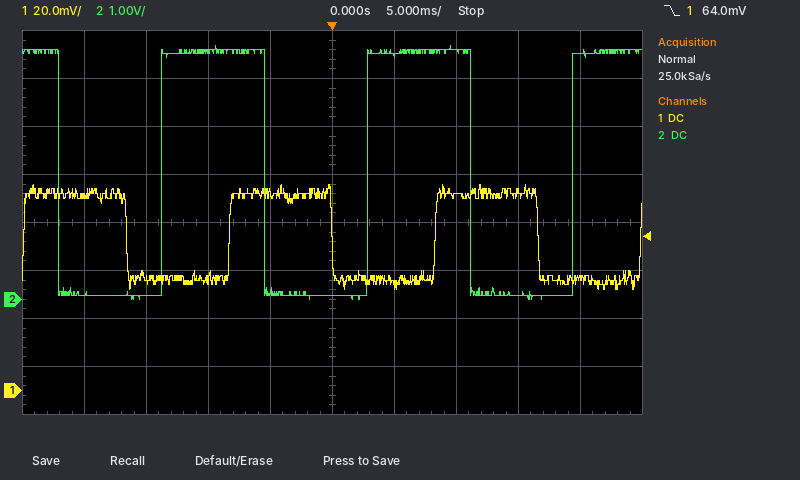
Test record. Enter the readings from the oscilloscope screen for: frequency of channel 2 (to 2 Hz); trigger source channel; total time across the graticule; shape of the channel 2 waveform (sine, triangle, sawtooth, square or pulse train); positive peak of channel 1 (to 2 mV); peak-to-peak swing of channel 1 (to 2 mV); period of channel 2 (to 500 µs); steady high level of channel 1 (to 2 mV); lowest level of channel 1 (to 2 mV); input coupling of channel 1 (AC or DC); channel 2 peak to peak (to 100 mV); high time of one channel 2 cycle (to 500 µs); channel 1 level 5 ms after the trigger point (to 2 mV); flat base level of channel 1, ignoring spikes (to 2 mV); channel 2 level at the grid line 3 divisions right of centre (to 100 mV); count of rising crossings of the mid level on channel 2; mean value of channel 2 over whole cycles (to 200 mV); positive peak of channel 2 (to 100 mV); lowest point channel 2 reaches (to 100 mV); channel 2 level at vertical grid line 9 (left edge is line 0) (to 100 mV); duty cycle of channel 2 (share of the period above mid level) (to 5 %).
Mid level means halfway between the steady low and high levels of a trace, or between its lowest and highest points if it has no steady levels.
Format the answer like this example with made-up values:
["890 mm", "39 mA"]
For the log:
["60 Hz", "channel 1", "50 ms", "square", "86 mV", "44 mV", "16.5 ms", "82 mV", "42 mV", "DC", "5.3 V", "8.5 ms", "44 mV", "46 mV", "100 mV", "3", "2.6 V", "5.3 V", "0.0 V", "5.1 V", "50 %"]
